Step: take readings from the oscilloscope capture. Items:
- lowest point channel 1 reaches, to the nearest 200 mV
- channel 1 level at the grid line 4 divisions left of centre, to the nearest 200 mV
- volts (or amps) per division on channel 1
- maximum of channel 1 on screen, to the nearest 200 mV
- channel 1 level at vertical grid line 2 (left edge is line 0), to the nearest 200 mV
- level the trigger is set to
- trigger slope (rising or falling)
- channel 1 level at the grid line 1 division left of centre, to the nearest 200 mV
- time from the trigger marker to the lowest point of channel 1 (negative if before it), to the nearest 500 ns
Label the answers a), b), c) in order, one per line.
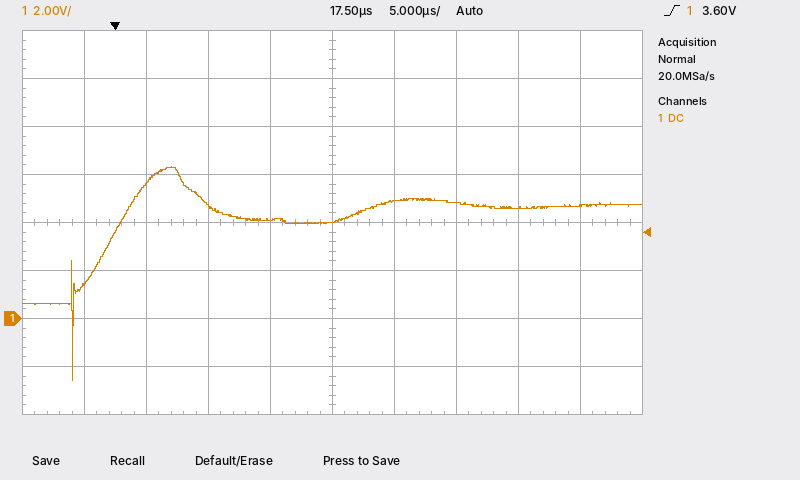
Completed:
a) -2.6 V
b) 1.4 V
c) 2 V
d) 6.4 V
e) 5.6 V
f) 3.60 V
g) rising
h) 4.2 V
i) -3.5 µs
